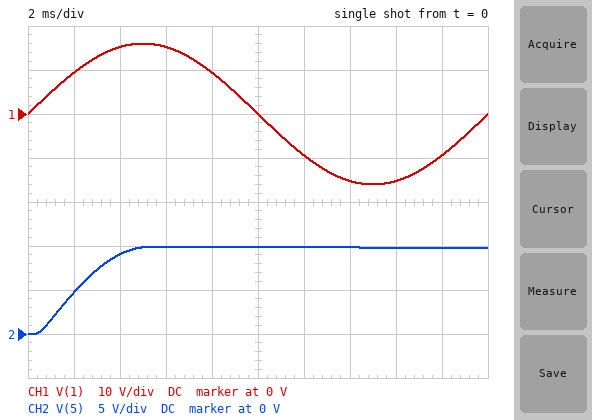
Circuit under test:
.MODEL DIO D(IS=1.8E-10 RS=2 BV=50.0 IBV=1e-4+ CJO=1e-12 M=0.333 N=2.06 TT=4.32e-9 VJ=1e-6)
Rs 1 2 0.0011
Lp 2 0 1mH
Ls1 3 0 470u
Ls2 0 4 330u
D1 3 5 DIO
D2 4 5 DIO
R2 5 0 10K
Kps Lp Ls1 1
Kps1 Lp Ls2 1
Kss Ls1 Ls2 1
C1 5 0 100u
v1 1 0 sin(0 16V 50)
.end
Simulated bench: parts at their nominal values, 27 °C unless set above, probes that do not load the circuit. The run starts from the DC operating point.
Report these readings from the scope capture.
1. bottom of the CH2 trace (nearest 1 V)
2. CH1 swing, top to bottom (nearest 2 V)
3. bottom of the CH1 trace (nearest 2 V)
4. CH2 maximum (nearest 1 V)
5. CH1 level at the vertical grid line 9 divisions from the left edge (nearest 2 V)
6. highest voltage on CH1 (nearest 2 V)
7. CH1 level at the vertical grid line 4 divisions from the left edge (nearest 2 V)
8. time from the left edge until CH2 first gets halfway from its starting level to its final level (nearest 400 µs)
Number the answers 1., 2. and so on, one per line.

1. 0 V
2. 32 V
3. -16 V
4. 10 V
5. -10 V
6. 16 V
7. 10 V
8. 2.0 ms
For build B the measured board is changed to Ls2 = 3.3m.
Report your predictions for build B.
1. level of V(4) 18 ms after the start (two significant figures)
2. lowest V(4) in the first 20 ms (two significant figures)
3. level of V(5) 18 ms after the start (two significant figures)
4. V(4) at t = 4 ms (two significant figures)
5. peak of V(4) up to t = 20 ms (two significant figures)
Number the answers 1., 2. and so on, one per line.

1. 17 V
2. -29 V
3. 28 V
4. -28 V
5. 29 V
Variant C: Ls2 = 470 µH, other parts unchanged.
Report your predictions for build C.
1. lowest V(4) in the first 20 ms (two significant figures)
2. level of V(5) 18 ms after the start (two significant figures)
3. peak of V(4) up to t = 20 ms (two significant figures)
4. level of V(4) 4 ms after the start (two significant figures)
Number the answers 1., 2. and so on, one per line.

1. -11 V
2. 10 V
3. 11 V
4. -10 V
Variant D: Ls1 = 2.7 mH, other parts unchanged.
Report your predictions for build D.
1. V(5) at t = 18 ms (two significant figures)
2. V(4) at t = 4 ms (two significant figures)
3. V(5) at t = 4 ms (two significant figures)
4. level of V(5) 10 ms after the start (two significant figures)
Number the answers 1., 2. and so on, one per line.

1. 24 V
2. -8.7 V
3. 23 V
4. 25 V
